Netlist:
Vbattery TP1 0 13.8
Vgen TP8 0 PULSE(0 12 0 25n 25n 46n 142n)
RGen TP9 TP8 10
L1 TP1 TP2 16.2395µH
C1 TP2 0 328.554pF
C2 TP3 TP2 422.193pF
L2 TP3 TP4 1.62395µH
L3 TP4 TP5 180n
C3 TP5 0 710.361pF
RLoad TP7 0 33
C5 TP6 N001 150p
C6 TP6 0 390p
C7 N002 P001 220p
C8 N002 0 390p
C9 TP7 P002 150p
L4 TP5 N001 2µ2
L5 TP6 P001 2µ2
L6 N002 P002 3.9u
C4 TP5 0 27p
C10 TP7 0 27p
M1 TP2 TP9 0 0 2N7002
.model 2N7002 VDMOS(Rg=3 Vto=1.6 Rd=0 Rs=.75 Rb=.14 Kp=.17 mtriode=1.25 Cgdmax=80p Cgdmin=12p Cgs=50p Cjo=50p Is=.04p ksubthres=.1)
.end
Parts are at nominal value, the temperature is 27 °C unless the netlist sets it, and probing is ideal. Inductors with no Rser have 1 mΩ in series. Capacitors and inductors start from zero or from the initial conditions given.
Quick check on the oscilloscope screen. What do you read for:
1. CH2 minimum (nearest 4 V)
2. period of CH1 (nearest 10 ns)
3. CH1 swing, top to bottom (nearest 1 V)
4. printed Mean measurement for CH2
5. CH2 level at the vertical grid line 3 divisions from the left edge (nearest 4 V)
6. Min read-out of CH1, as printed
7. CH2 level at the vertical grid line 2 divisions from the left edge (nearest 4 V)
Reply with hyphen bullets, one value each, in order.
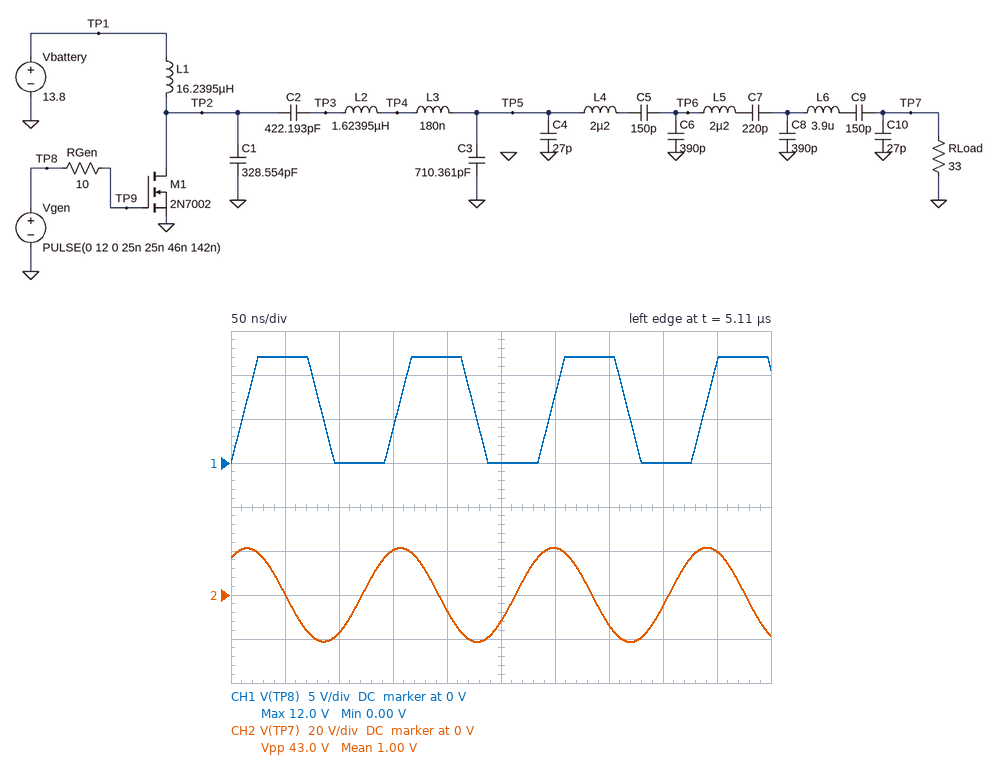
- -20 V
- 140 ns
- 12 V
- 1.00 V
- 20 V
- 0.00 V
- -16 V
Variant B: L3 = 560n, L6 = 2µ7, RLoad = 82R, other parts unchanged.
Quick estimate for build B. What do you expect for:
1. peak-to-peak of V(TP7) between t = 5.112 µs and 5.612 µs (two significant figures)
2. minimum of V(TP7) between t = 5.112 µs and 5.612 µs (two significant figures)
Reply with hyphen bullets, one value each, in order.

- 16 V
- -7.8 V
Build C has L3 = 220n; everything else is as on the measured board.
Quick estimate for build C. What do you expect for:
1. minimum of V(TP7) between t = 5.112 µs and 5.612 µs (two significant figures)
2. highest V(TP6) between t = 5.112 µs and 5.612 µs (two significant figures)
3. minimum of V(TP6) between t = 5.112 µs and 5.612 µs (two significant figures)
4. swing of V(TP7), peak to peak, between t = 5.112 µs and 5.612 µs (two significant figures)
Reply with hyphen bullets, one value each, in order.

- -22 V
- 28 V
- -27 V
- 44 V
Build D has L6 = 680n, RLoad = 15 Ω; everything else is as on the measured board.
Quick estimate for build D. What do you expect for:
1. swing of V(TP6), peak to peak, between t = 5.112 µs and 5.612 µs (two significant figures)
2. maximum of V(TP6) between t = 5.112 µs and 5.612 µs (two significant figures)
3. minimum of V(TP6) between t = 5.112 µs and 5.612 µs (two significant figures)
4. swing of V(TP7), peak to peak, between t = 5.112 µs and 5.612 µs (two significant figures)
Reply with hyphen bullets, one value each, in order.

- 46 V
- 24 V
- -22 V
- 5.0 V
